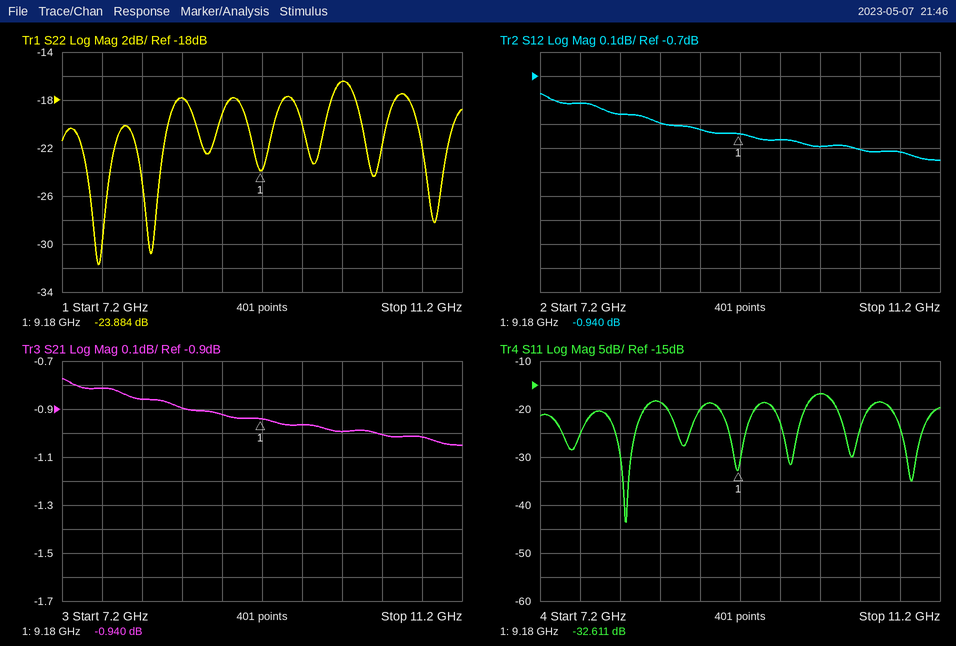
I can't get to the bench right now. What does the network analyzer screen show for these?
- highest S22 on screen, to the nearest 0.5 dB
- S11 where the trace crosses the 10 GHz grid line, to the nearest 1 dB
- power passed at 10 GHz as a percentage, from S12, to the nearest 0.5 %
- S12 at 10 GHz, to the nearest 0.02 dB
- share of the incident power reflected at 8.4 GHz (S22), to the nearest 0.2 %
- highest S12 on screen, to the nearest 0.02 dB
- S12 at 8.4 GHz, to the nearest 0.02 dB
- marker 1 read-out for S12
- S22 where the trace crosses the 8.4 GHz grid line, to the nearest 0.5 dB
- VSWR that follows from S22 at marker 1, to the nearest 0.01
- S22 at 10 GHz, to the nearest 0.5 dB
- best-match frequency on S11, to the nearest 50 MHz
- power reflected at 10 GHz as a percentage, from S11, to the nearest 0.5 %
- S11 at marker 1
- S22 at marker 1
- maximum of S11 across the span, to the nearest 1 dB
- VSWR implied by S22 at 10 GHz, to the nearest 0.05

-16.5 dB
-17 dB
79.5 %
-1.00 dB
1.6 %
-0.78 dB
-0.90 dB
-0.940 dB
-18.0 dB
1.14
-16.5 dB
8.05 GHz
2.0 %
-32.611 dB
-23.884 dB
-17 dB
1.35
